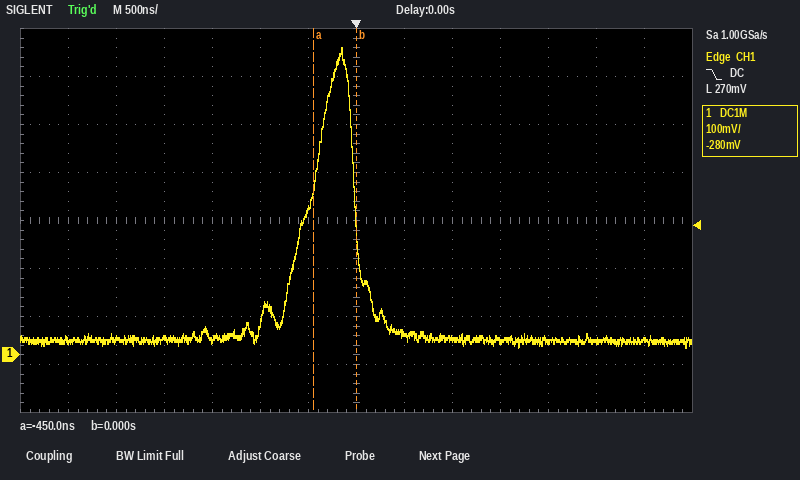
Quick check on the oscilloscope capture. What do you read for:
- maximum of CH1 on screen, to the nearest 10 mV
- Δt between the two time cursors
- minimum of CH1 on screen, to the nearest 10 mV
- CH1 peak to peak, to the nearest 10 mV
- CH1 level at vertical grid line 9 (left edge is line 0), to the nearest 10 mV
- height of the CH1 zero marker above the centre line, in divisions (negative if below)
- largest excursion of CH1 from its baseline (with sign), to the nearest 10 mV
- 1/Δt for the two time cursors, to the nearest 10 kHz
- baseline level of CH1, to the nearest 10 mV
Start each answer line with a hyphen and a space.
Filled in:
- 640 mV
- 450 ns
- 20 mV
- 620 mV
- 30 mV
- -2.8 div
- +610 mV
- 2.22 MHz
- 30 mV
